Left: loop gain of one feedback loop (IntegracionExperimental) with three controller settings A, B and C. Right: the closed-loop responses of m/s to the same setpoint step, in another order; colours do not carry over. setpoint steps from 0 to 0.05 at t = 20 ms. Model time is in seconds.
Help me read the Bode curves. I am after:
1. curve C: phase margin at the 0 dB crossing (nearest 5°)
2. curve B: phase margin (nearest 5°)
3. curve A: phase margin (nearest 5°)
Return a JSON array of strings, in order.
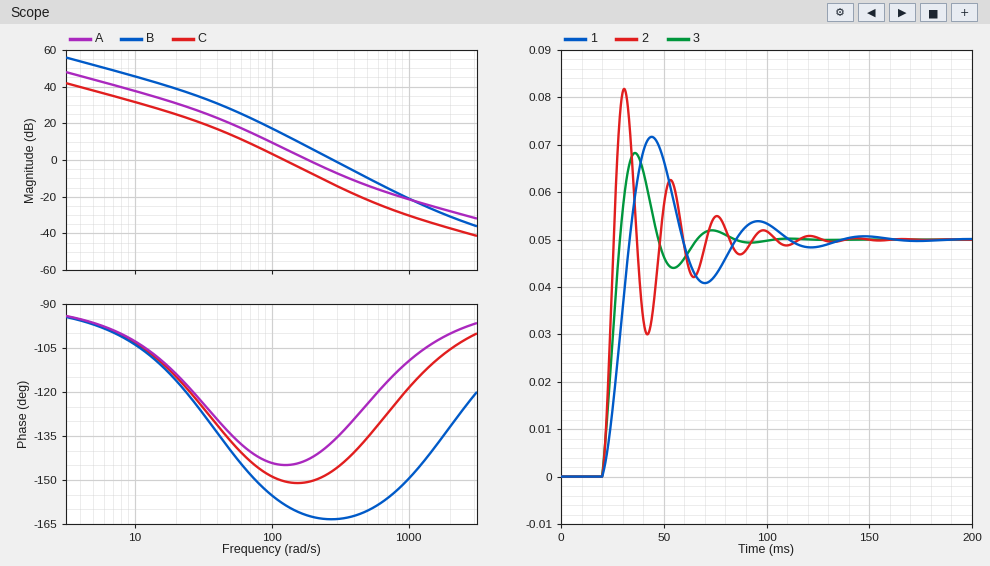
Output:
["30°", "15°", "35°"]
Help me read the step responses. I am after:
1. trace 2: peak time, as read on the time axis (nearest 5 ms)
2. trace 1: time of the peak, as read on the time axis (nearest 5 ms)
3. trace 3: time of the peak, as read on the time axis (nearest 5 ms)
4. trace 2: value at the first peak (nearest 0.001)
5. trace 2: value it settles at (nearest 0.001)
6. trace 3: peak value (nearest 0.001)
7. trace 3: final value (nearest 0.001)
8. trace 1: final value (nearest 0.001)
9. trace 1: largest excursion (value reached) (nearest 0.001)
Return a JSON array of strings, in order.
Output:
["30 ms", "45 ms", "35 ms", "0.082", "0.050", "0.068", "0.050", "0.050", "0.072"]
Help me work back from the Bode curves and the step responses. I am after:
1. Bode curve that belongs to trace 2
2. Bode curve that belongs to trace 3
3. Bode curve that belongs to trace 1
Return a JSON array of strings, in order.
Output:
["B", "A", "C"]
